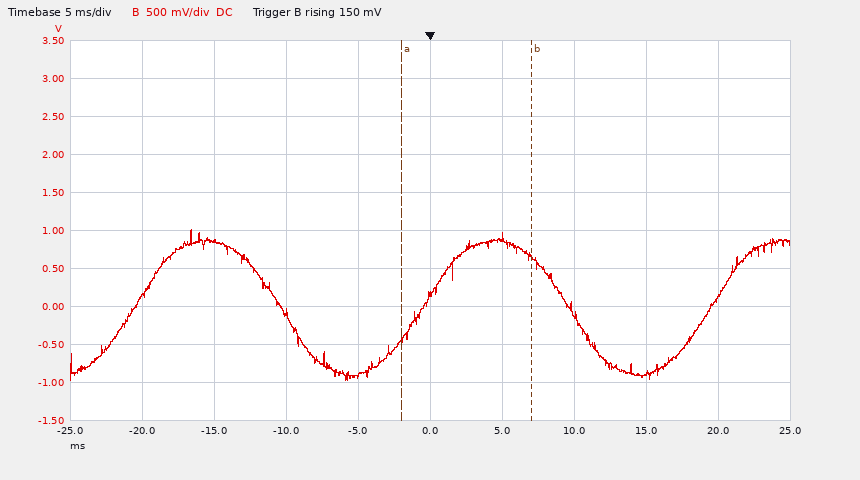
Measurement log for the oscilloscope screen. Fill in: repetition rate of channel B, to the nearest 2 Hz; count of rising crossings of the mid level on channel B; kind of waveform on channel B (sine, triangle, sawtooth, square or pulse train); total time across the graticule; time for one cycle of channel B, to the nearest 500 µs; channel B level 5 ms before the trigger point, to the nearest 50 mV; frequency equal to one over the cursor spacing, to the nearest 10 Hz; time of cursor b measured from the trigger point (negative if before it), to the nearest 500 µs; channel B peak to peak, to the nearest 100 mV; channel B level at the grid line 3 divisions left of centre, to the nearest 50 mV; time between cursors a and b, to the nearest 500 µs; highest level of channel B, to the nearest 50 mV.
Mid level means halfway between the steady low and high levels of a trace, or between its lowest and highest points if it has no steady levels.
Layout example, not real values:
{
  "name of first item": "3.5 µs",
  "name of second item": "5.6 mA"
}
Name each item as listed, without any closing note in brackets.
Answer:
{
  "repetition rate of channel B, to the nearest 2 Hz": "50 Hz",
  "count of rising crossings of the mid level on channel B": "3",
  "kind of waveform on channel B": "sine",
  "total time across the graticule": "50 ms",
  "time for one cycle of channel B, to the nearest 500 µs": "20.0 ms",
  "channel B level 5 ms before the trigger point, to the nearest 50 mV": "-900 mV",
  "frequency equal to one over the cursor spacing, to the nearest 10 Hz": "110 Hz",
  "time of cursor b measured from the trigger point (negative if before it), to the nearest 500 µs": "+7.0 ms",
  "channel B peak to peak, to the nearest 100 mV": "2.00 V",
  "channel B level at the grid line 3 divisions left of centre, to the nearest 50 mV": "850 mV",
  "time between cursors a and b, to the nearest 500 µs": "9.0 ms",
  "highest level of channel B, to the nearest 50 mV": "1.00 V"
}
